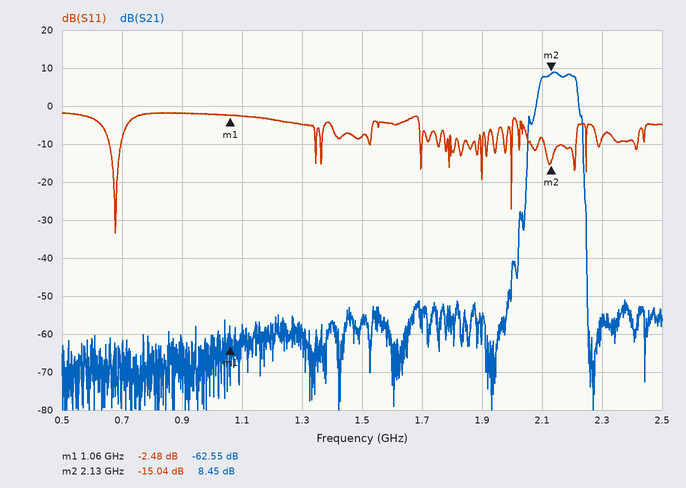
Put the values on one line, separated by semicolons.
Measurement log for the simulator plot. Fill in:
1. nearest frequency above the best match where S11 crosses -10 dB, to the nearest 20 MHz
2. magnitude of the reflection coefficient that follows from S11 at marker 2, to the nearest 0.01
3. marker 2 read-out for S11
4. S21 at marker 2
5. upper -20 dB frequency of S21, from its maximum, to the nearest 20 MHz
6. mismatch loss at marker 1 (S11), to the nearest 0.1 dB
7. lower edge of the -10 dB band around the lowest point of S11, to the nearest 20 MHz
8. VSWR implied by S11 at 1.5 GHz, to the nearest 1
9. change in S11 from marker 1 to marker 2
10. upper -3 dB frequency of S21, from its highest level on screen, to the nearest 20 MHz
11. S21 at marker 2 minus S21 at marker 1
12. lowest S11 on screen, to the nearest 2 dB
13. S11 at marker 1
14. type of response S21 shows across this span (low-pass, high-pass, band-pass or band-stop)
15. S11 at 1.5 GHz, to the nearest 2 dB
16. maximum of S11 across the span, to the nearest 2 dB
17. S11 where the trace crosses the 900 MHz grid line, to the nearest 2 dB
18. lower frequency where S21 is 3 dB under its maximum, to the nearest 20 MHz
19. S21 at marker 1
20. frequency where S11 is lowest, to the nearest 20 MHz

700 MHz; 0.18; -15.04 dB; 8.45 dB; 2.24 GHz; 3.6 dB; 660 MHz; 2; -12.56 dB; 2.22 GHz; 71.00 dB; -34 dB; -2.48 dB; band-pass; -8 dB; -2 dB; -2 dB; 2.10 GHz; -62.55 dB; 680 MHz
